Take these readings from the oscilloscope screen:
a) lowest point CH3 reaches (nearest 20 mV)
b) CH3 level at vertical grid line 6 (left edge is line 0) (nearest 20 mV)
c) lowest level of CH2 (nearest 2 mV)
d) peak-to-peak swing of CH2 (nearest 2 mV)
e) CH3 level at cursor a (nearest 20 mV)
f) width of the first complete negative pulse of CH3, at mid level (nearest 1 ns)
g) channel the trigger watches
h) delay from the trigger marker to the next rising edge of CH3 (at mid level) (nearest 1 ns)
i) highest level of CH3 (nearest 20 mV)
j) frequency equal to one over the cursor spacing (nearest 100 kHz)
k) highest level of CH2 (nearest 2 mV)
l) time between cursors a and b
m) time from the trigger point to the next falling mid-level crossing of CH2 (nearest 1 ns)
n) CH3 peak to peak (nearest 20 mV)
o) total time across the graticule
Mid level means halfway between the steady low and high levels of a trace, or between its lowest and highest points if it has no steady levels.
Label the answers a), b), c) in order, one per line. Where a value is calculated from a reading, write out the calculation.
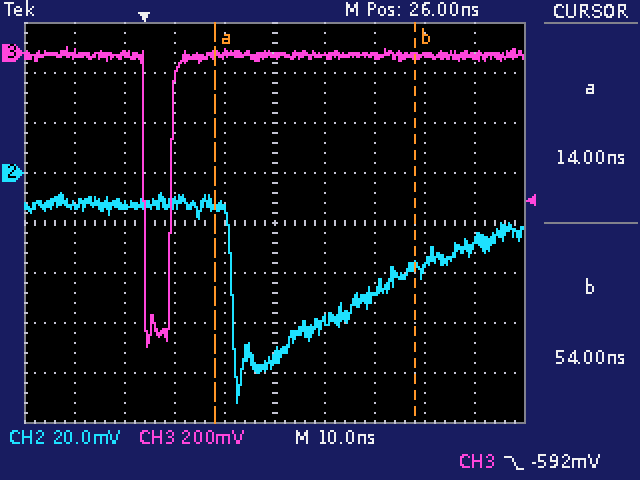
a) -1.18 V
b) -20 mV
c) -92 mV
d) -8 mV − (-92 mV) = 84 mV
e) 0 mV
f) 5 ns
g) CH3
h) 5 ns
i) 20 mV
j) 1 / 40 ns ≈ 25.0 MHz
k) -8 mV
l) 54 ns − (14 ns) = 40 ns
m) 18 ns
n) 20 mV − (-1.18 V) = 1.20 V
o) 100 ns
